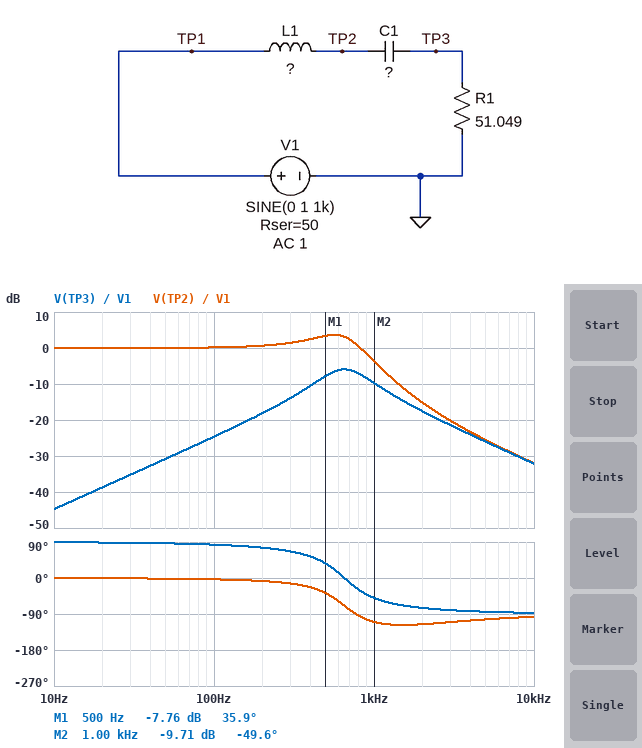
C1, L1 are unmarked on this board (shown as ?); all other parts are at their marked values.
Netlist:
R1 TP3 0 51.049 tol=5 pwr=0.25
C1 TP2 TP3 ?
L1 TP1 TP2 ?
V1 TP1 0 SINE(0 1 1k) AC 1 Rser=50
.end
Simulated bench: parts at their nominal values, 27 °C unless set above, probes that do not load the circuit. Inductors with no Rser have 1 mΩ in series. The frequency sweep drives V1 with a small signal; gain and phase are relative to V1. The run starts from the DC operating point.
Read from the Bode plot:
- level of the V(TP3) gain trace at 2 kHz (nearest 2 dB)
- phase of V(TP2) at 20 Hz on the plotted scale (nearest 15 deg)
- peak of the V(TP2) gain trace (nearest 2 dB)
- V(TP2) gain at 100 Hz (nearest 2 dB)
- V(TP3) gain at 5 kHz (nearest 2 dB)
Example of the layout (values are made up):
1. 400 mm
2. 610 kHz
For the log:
1. -18 dB
2. 0 deg
3. 4 dB
4. 0 dB
5. -26 dB
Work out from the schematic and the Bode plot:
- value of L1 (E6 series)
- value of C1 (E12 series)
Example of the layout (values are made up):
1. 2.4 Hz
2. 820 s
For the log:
1. 33 mH
2. 1.8 µF
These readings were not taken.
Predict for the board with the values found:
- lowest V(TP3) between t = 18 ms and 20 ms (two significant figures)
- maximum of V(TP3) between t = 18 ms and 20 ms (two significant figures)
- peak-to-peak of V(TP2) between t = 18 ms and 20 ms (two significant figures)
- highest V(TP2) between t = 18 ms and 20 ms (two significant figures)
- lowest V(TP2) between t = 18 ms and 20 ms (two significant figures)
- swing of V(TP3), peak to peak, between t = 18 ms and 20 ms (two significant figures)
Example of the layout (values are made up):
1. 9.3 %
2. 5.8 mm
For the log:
1. -330 mV
2. 330 mV
3. 1.3 V
4. 650 mV
5. -650 mV
6. 650 mV
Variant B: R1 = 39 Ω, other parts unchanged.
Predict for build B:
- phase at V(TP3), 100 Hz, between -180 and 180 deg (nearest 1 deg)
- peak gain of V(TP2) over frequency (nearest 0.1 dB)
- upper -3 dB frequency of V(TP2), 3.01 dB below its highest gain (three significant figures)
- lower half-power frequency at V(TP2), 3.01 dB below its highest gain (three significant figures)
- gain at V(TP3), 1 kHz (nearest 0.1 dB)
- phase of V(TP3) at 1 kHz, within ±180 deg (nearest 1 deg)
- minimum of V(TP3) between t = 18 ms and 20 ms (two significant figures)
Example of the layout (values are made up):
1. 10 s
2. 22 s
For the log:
1. 84 deg
2. 4.4 dB
3. 782 Hz
4. 287 Hz
5. -11.6 dB
6. -53 deg
7. -260 mV
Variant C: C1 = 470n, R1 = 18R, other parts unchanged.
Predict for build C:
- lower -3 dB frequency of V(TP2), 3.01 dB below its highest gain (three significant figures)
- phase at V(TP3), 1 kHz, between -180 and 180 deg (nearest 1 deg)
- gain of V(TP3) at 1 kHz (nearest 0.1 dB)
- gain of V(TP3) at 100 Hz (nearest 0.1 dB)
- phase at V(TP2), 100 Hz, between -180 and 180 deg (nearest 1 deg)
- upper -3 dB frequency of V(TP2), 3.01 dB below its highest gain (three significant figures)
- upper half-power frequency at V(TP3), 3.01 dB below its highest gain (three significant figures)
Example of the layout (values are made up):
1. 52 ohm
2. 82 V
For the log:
1. 1.08 kHz
2. 63 deg
3. -18.3 dB
4. -45.4 dB
5. -1 deg
6. 1.41 kHz
7. 1.45 kHz
